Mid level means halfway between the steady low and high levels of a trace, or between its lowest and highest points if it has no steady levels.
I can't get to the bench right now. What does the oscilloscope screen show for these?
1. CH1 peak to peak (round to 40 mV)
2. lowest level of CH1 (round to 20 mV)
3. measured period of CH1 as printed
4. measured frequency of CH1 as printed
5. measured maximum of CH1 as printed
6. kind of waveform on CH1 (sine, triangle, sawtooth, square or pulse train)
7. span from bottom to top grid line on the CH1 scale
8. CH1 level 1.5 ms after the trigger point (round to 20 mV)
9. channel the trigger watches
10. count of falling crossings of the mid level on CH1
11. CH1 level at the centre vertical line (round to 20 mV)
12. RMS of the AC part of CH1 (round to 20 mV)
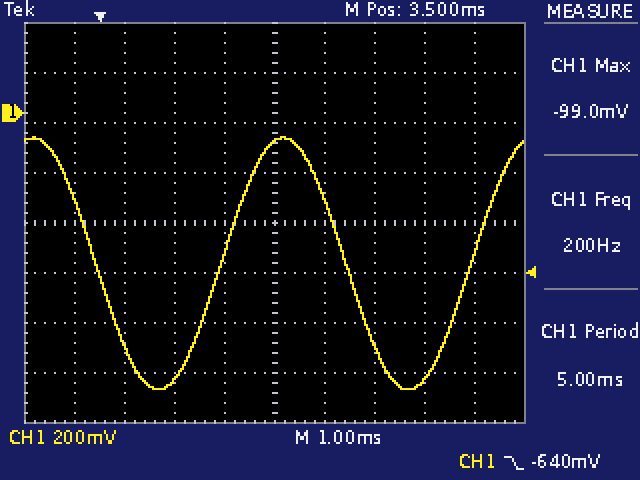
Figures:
1.00 V
-1.10 V
5.00 ms
200 Hz
-99.0 mV
sine
1.6 V
-1.06 V
CH1
2
-120 mV
360 mV
